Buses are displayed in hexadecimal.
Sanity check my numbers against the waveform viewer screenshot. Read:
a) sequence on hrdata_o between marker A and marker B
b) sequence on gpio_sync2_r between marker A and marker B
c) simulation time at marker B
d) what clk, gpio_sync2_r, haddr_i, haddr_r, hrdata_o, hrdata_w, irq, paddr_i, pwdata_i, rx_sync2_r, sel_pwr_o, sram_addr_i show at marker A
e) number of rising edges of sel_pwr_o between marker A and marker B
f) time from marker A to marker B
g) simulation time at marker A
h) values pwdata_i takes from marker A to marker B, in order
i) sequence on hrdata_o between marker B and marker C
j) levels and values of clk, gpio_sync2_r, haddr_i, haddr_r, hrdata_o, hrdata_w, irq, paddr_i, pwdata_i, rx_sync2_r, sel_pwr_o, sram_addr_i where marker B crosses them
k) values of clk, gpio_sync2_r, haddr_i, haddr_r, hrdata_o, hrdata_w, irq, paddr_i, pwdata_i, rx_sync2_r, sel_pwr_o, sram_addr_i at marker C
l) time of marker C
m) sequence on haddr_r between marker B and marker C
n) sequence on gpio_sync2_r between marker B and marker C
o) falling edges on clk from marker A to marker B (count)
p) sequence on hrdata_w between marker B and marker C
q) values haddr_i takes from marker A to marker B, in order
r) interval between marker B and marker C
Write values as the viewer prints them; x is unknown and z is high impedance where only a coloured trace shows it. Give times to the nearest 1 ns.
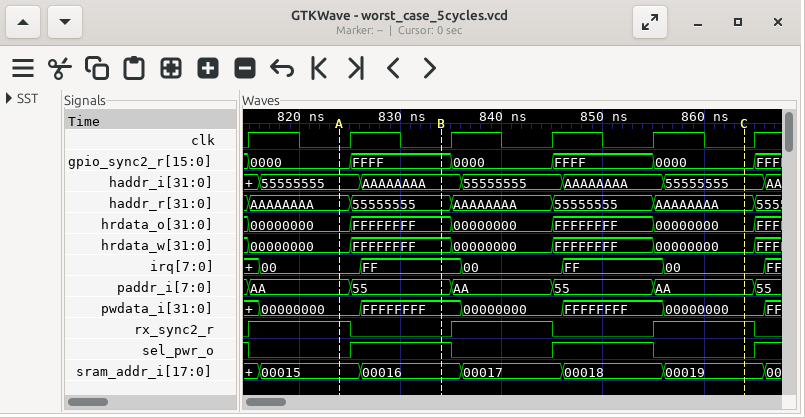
00000000, FFFFFFFF
0000, FFFF
834 ns
clk=0, gpio_sync2_r=0000, haddr_i=55555555, haddr_r=AAAAAAAA, hrdata_o=00000000, hrdata_w=00000000, irq=00, paddr_i=AA, pwdata_i=00000000, rx_sync2_r=1, sel_pwr_o=0, sram_addr_i=00015
1
10 ns
824 ns
00000000, FFFFFFFF
FFFFFFFF, 00000000, FFFFFFFF, 00000000
clk=0, gpio_sync2_r=FFFF, haddr_i=AAAAAAAA, haddr_r=55555555, hrdata_o=FFFFFFFF, hrdata_w=FFFFFFFF, irq=FF, paddr_i=55, pwdata_i=FFFFFFFF, rx_sync2_r=0, sel_pwr_o=1, sram_addr_i=00016
clk=0, gpio_sync2_r=0000, haddr_i=55555555, haddr_r=AAAAAAAA, hrdata_o=00000000, hrdata_w=00000000, irq=00, paddr_i=AA, pwdata_i=00000000, rx_sync2_r=1, sel_pwr_o=0, sram_addr_i=00019
864 ns
55555555, AAAAAAAA, 55555555, AAAAAAAA
FFFF, 0000, FFFF, 0000
1
FFFFFFFF, 00000000, FFFFFFFF, 00000000
55555555, AAAAAAAA
30 ns
